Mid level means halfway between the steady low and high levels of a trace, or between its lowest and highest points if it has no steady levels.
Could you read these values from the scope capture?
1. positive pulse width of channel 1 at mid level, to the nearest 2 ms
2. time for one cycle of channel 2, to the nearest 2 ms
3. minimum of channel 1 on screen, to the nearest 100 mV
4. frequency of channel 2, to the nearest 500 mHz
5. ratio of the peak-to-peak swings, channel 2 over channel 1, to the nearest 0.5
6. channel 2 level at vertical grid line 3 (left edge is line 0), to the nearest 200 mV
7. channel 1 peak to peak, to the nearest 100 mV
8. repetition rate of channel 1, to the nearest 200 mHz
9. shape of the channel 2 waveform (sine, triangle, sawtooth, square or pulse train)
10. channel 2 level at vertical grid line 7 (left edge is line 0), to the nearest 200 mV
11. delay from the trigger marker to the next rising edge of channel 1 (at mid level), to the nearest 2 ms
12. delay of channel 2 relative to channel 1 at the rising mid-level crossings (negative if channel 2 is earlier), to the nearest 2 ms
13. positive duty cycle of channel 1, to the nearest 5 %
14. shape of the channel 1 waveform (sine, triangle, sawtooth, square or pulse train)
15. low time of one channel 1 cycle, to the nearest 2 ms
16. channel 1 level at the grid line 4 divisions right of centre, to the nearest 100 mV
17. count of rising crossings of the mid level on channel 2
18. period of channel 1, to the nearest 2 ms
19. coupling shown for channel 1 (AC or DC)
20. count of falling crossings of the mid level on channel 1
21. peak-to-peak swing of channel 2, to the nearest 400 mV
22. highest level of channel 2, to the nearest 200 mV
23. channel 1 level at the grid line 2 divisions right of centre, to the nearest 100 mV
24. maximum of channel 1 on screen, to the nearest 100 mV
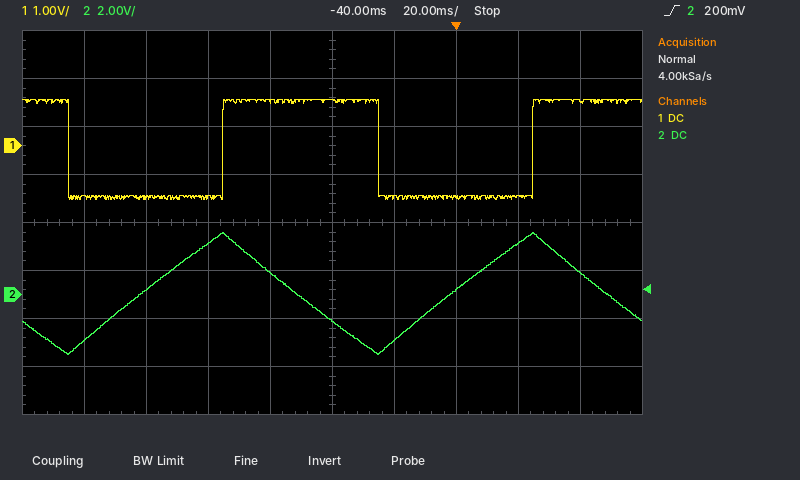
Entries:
50 ms
100 ms
-1.1 V
10.0 Hz
2.5
2.2 V
2.1 V
10.0 Hz
triangle
200 mV
24 ms
-26 ms
50 %
square
50 ms
900 mV
2
100 ms
DC
2
5.2 V
2.6 V
-1.1 V
1.0 V
